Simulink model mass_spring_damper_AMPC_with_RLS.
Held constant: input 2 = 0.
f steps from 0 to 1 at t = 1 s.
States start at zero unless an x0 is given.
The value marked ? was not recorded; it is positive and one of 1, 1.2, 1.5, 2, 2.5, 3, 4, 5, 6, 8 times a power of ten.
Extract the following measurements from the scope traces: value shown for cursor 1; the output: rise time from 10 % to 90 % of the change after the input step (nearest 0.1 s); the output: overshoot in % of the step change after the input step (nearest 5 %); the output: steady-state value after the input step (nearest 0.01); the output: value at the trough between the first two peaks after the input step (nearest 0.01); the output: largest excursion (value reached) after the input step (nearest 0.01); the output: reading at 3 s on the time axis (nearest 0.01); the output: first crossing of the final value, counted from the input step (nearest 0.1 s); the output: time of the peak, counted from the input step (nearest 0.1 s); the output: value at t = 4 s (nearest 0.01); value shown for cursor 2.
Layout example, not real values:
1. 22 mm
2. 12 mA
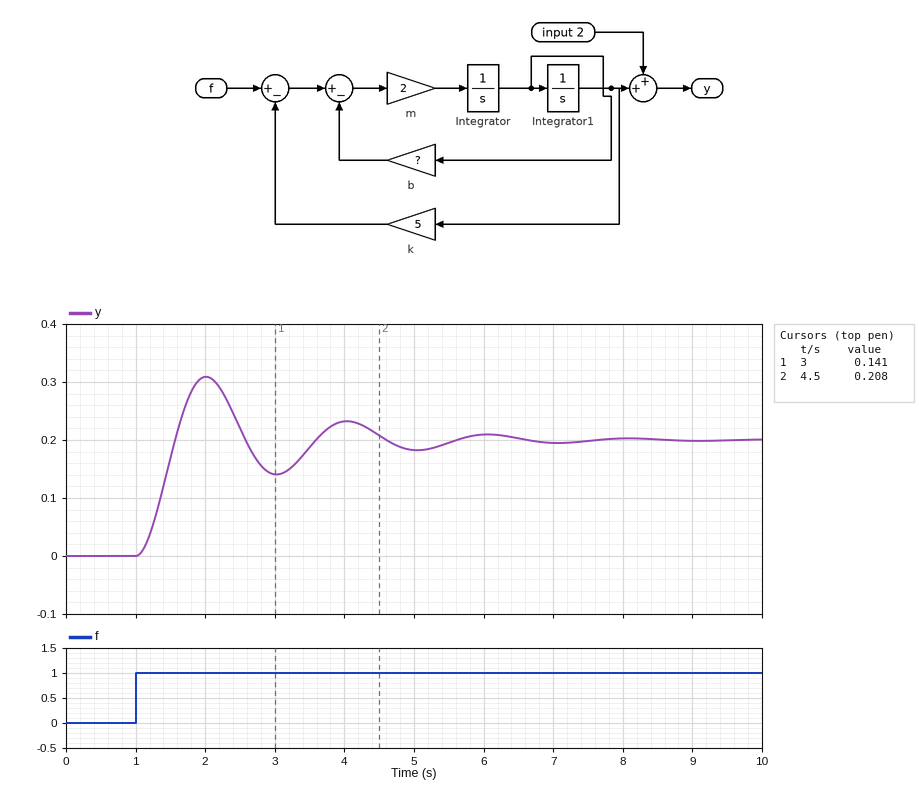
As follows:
1. 0.141
2. 0.4 s
3. 55 %
4. 0.20
5. 0.14
6. 0.31
7. 0.14
8. 0.6 s
9. 1.0 s
10. 0.23
11. 0.208
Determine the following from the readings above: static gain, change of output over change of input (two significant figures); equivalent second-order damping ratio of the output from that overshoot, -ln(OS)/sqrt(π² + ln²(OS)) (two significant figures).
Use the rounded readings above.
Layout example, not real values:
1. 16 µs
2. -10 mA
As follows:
1. 0.20
2. 0.19
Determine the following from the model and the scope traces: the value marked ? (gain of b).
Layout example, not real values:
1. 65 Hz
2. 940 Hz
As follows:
1. 0.6
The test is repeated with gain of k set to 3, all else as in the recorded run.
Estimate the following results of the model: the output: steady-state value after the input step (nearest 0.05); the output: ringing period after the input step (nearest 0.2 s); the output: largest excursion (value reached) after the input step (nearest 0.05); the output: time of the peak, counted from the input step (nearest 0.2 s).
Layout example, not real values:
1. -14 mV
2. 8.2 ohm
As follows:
1. 0.35
2. 2.6 s
3. 0.50
4. 1.4 s
